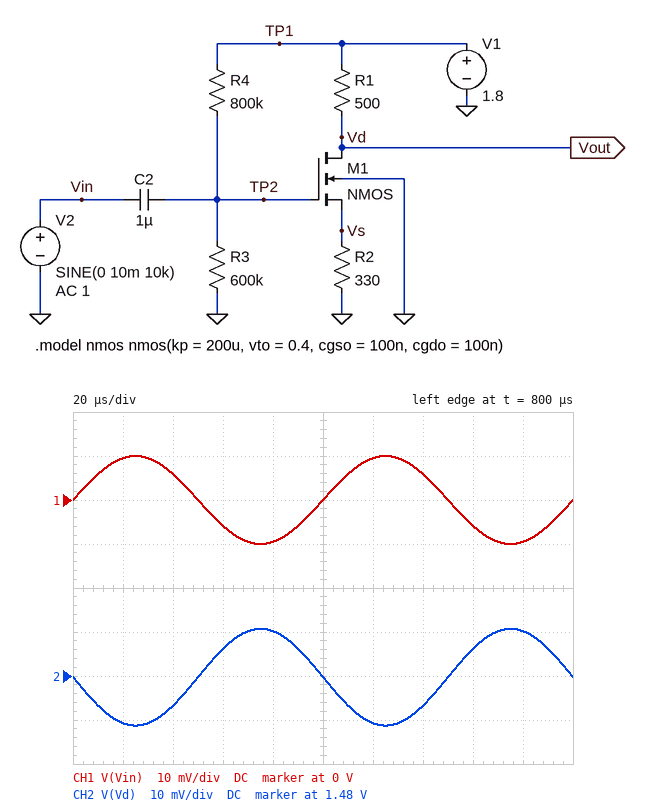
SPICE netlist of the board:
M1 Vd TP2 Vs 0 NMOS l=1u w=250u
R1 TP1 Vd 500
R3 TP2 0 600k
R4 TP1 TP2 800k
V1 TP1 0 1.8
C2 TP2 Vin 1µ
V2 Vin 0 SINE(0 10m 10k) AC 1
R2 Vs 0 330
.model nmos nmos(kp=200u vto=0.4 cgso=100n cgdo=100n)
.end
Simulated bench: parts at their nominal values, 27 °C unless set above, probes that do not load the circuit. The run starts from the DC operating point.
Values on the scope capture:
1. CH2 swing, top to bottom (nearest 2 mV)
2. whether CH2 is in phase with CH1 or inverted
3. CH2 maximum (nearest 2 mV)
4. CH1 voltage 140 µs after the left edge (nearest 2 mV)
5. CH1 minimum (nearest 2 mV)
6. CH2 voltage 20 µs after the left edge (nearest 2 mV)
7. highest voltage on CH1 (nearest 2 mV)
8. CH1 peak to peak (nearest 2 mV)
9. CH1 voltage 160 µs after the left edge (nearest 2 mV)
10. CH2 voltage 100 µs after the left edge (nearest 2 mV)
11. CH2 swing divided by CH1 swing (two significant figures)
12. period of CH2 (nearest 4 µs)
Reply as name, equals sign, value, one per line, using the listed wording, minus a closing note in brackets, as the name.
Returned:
CH2 swing, top to bottom = 22 mV
whether CH2 is in phase with CH1 or inverted = inverted
CH2 maximum = 1.490 V
CH1 voltage 140 µs after the left edge = 6 mV
CH1 minimum = -10 mV
CH2 voltage 20 µs after the left edge = 1.470 V
highest voltage on CH1 = 10 mV
CH1 peak to peak = 20 mV
CH1 voltage 160 µs after the left edge = -6 mV
CH2 voltage 100 µs after the left edge = 1.480 V
CH2 swing divided by CH1 swing = 1.1
period of CH2 = 100 µs
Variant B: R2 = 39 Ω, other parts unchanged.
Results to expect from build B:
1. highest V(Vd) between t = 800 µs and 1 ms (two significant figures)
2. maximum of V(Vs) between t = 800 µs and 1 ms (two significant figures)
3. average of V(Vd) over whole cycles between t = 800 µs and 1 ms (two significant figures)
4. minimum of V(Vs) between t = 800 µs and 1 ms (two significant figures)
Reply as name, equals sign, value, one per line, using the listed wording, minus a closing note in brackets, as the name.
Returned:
highest V(Vd) between t = 800 µs and 1 ms = 800 mV
maximum of V(Vs) between t = 800 µs and 1 ms = 85 mV
average of V(Vd) over whole cycles between t = 800 µs and 1 ms = 750 mV
minimum of V(Vs) between t = 800 µs and 1 ms = 78 mV
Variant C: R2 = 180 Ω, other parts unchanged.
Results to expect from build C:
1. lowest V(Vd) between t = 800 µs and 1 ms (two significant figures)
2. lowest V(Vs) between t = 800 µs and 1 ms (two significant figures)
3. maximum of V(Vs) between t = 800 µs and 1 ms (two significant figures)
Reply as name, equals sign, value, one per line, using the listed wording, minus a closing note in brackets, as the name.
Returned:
lowest V(Vd) between t = 800 µs and 1 ms = 1.3 V
lowest V(Vs) between t = 800 µs and 1 ms = 170 mV
maximum of V(Vs) between t = 800 µs and 1 ms = 180 mV
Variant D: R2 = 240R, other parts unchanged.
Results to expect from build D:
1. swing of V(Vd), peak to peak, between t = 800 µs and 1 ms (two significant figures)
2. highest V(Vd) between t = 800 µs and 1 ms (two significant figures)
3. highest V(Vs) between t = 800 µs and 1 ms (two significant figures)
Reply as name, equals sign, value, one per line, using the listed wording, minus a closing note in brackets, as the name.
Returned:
swing of V(Vd), peak to peak, between t = 800 µs and 1 ms = 28 mV
highest V(Vd) between t = 800 µs and 1 ms = 1.4 V
highest V(Vs) between t = 800 µs and 1 ms = 200 mV
